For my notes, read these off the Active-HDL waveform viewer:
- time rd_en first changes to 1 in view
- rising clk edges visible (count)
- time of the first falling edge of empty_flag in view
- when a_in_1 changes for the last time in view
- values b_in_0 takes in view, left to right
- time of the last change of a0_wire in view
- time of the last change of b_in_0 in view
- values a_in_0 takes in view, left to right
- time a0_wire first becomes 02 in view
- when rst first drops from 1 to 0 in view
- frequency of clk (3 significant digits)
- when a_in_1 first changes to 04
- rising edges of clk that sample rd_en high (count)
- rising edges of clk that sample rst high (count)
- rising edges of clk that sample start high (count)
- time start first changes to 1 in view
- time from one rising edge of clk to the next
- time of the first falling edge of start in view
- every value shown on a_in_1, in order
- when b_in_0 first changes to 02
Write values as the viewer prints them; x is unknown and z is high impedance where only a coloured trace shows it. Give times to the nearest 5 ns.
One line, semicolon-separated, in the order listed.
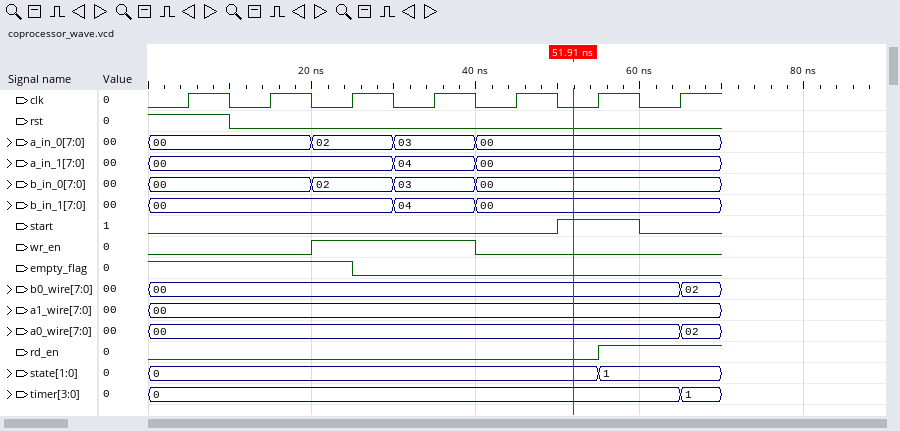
55 ns; 7; 25 ns; 40 ns; 00, 02, 03, 00; 65 ns; 40 ns; 00, 02, 03, 00; 65 ns; 10 ns; 100 MHz; 30 ns; 1; 1; 1; 50 ns; 10 ns; 60 ns; 00, 04, 00; 20 ns
